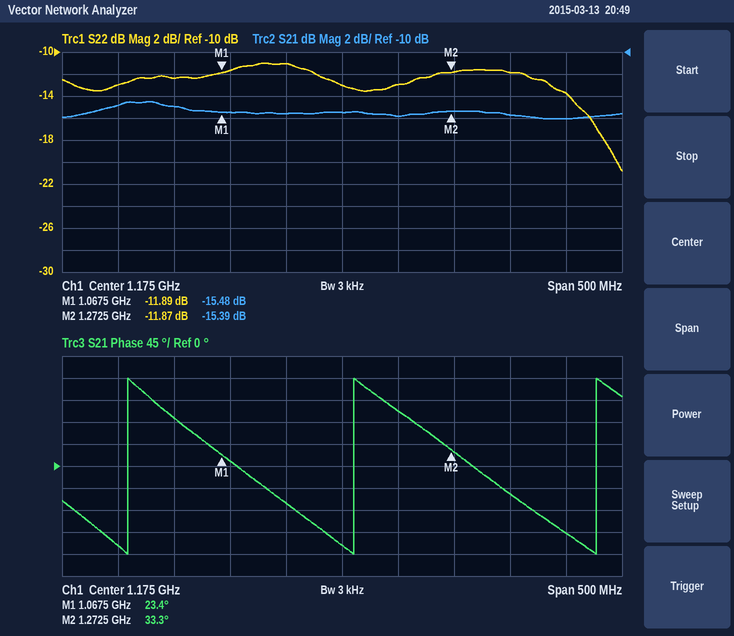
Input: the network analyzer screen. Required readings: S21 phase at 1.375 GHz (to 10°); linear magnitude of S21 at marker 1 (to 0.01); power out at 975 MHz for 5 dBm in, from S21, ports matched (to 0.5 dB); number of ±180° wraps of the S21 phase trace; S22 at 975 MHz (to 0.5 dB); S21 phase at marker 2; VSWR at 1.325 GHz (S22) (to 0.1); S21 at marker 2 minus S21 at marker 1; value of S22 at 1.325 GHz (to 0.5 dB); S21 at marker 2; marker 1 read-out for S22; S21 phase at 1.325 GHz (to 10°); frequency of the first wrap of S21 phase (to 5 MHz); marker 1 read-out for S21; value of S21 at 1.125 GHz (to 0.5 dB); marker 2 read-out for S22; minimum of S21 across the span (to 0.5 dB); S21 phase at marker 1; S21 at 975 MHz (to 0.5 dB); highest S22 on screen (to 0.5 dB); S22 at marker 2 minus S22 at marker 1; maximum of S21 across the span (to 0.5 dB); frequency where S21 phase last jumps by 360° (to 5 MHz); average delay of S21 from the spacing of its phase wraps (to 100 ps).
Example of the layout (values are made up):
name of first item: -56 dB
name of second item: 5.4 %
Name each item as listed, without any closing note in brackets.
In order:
S21 phase at 1.375 GHz: -140°
linear magnitude of S21 at marker 1: 0.17
power out at 975 MHz for 5 dBm in, from S21, ports matched: -10.0 dBm
number of ±180° wraps of the S21 phase trace: 3
S22 at 975 MHz: -13.0 dB
S21 phase at marker 2: 33.3°
VSWR at 1.325 GHz (S22): 1.7
S21 at marker 2 minus S21 at marker 1: 0.09 dB
value of S22 at 1.325 GHz: -12.0 dB
S21 at marker 2: -15.39 dB
marker 1 read-out for S22: -11.89 dB
S21 phase at 1.325 GHz: -60°
frequency of the first wrap of S21 phase: 985 MHz
marker 1 read-out for S21: -15.48 dB
value of S21 at 1.125 GHz: -15.5 dB
marker 2 read-out for S22: -11.87 dB
minimum of S21 across the span: -16.0 dB
S21 phase at marker 1: 23.4°
S21 at 975 MHz: -15.0 dB
highest S22 on screen: -11.0 dB
S22 at marker 2 minus S22 at marker 1: 0.02 dB
maximum of S21 across the span: -14.5 dB
frequency where S21 phase last jumps by 360°: 1.400 GHz
average delay of S21 from the spacing of its phase wraps: 4.8 ns
